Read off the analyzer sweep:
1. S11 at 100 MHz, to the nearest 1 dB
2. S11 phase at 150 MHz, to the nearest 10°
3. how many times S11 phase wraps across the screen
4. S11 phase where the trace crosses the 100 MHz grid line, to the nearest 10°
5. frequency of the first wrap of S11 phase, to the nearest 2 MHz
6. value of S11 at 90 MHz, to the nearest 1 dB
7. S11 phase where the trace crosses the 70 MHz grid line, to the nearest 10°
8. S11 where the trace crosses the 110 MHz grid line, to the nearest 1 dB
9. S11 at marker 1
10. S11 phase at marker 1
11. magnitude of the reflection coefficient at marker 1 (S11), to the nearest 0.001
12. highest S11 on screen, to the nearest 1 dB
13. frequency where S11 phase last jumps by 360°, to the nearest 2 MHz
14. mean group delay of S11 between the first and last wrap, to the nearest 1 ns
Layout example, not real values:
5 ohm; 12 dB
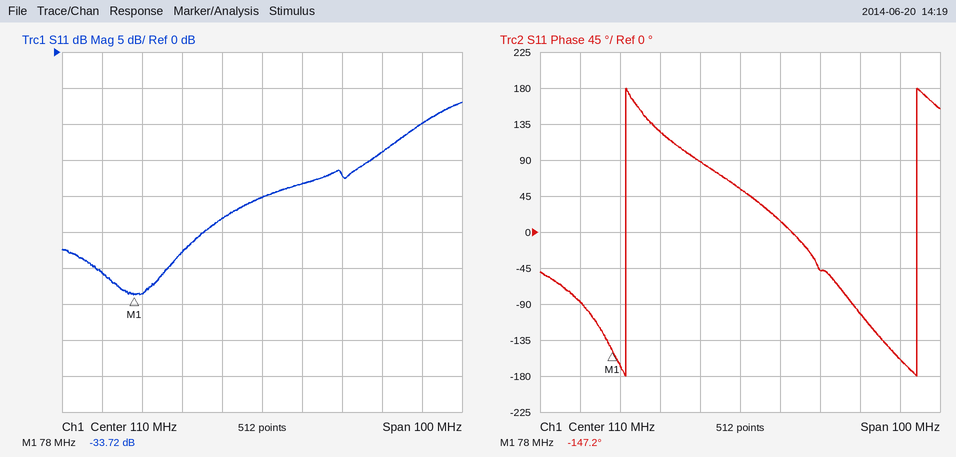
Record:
-23 dB; -160°; 2; 90°; 82 MHz; -28 dB; -90°; -20 dB; -33.72 dB; -147.2°; 0.021; -7 dB; 154 MHz; 14 ns
